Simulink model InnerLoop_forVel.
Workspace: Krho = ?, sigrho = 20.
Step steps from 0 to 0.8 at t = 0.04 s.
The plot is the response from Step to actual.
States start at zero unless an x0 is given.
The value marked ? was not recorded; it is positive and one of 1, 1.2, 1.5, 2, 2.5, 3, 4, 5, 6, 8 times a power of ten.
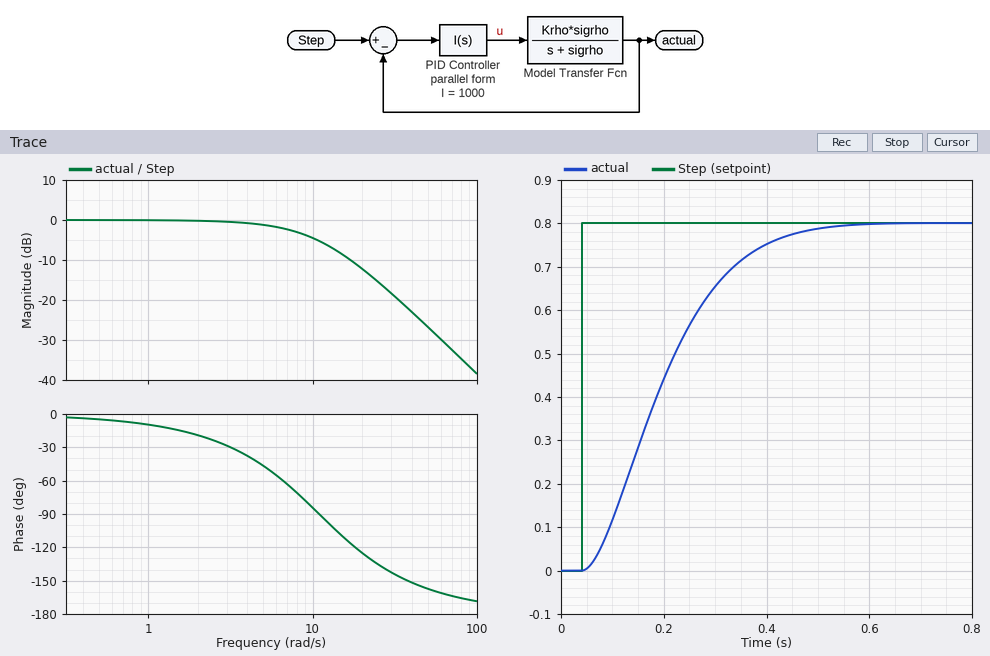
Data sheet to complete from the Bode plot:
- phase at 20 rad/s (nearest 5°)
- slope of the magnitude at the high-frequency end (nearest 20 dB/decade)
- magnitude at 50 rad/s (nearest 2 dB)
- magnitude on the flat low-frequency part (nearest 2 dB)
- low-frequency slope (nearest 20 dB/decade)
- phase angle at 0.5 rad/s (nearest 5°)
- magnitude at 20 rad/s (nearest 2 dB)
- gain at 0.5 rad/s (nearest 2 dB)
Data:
-125°
-40 dB/decade
-26 dB
0 dB
0 dB/decade
-5°
-12 dB
0 dB
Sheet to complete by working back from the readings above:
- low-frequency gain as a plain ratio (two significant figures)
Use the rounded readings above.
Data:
1.0
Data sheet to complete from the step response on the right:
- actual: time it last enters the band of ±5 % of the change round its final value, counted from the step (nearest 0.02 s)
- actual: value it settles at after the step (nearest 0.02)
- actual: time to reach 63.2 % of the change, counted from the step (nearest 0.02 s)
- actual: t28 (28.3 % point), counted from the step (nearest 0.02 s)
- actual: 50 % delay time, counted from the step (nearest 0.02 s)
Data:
0.38 s
0.80
0.18 s
0.10 s
0.14 s
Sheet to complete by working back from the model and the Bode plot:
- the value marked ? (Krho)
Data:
0.006
